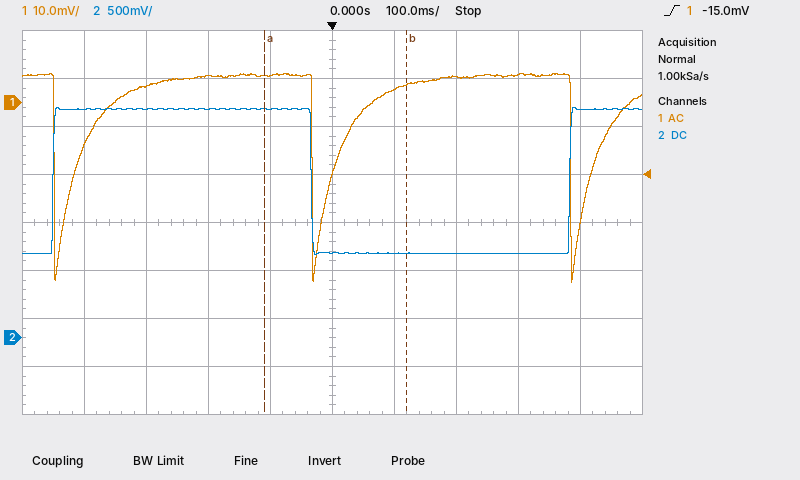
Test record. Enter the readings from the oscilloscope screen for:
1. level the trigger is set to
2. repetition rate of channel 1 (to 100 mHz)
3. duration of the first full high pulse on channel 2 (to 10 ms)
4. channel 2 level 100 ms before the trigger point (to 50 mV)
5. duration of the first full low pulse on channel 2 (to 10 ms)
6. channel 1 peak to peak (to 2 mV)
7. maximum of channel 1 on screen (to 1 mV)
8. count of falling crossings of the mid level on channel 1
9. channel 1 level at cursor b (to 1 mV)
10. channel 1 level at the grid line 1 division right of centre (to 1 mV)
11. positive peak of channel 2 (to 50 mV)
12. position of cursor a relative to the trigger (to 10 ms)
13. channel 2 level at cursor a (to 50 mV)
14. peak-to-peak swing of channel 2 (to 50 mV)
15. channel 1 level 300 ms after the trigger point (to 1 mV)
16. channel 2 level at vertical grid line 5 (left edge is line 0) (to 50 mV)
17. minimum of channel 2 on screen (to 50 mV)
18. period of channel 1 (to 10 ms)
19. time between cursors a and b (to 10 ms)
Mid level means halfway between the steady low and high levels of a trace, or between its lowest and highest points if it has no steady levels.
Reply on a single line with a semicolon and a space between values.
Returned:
-15.0 mV; 2.4 Hz; 420 ms; 2.40 V; 420 ms; 44 mV; 6 mV; 3; 4 mV; 3 mV; 2.40 V; -110 ms; 2.40 V; 1.55 V; 6 mV; 900 mV; 850 mV; 420 ms; 230 ms
